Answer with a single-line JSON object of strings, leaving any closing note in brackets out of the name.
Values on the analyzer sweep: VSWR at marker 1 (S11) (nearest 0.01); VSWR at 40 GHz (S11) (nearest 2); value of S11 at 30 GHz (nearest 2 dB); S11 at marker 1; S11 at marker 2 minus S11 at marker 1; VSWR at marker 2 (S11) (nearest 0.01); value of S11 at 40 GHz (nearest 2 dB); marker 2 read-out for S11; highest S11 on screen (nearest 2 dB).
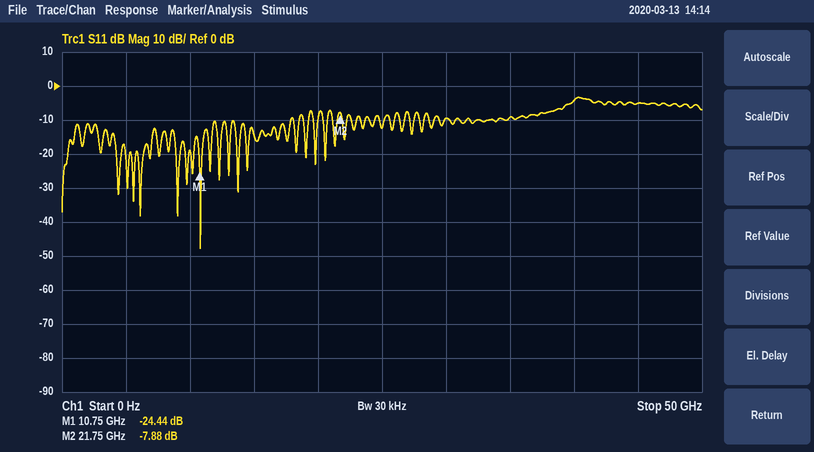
{"VSWR at marker 1 (S11)": "1.13", "VSWR at 40 GHz (S11)": "4", "value of S11 at 30 GHz": "-10 dB", "S11 at marker 1": "-24.44 dB", "S11 at marker 2 minus S11 at marker 1": "16.56 dB", "VSWR at marker 2 (S11)": "2.35", "value of S11 at 40 GHz": "-4 dB", "marker 2 read-out for S11": "-7.88 dB", "highest S11 on screen": "-4 dB"}
